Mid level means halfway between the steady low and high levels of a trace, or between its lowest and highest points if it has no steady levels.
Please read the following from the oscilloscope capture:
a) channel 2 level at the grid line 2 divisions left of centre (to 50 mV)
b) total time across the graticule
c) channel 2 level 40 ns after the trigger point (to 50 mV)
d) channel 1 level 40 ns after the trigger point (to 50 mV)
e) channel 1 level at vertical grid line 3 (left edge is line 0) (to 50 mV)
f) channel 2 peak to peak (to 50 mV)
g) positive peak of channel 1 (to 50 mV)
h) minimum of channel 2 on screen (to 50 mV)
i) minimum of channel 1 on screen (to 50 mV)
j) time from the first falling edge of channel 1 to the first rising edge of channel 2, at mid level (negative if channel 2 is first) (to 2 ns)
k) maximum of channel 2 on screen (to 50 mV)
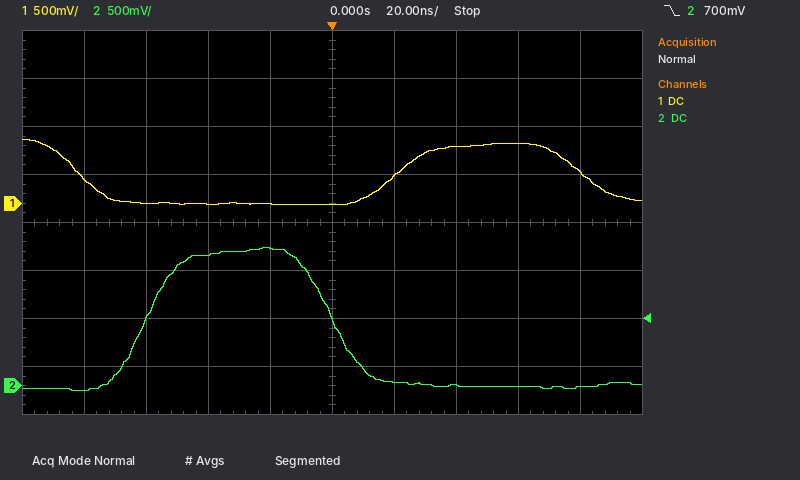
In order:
1.35 V
200 ns
0 mV
600 mV
0 mV
1.50 V
650 mV
-50 mV
0 mV
+22 ns
1.45 V
